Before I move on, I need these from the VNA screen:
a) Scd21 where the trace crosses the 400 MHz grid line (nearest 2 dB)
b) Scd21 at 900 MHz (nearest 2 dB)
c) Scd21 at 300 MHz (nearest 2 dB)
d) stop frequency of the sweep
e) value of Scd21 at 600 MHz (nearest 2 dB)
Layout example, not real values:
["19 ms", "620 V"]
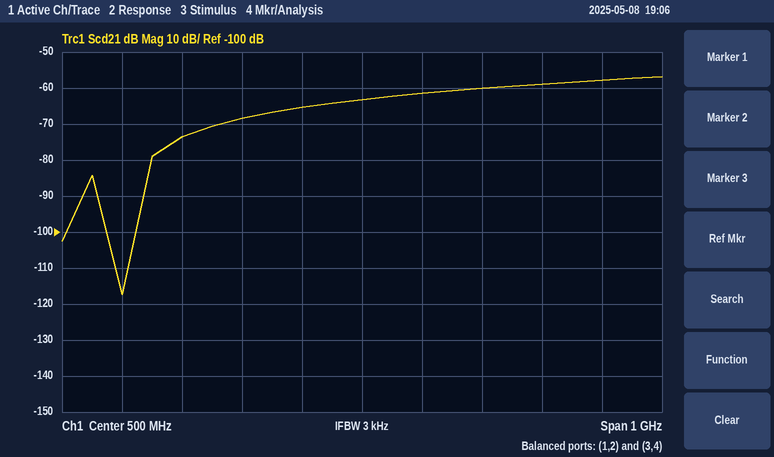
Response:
["-66 dB", "-58 dB", "-68 dB", "1 GHz", "-62 dB"]
